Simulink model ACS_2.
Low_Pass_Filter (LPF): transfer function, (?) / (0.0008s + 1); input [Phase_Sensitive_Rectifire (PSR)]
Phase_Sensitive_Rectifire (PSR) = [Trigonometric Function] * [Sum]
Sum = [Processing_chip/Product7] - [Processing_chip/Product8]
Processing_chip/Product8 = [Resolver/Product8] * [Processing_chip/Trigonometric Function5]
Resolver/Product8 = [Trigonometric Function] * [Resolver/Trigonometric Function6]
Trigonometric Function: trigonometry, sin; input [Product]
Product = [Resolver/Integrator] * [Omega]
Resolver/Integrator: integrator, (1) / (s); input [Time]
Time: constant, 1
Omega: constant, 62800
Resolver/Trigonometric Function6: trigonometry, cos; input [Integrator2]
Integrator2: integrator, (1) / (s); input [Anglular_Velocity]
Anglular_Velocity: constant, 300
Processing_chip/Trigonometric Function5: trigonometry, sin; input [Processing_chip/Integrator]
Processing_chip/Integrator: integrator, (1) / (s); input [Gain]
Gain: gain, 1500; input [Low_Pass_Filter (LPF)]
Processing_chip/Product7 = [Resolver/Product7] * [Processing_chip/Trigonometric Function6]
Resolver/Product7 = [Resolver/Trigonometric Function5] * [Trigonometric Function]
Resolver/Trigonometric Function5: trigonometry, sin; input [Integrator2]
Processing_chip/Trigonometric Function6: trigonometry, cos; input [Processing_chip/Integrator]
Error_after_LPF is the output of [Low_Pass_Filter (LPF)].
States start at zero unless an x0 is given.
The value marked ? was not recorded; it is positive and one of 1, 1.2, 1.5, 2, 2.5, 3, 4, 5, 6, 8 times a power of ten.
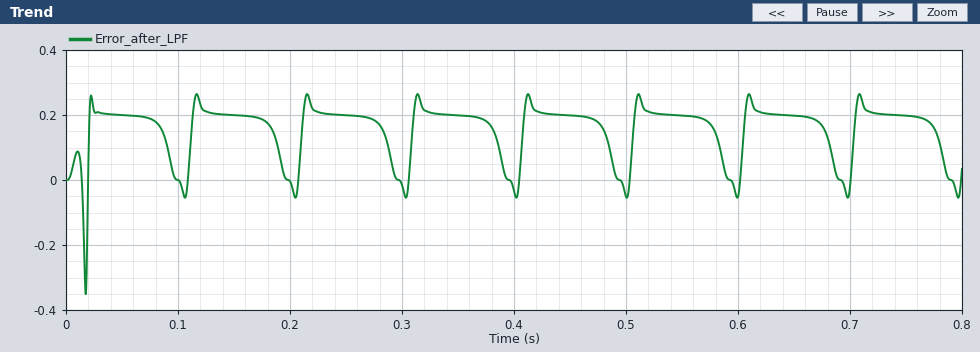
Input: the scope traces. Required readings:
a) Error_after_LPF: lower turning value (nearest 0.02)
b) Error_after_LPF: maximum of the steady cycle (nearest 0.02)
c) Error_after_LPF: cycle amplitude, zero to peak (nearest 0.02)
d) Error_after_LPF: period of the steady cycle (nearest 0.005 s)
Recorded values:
-0.06
0.26
0.16
0.100 s
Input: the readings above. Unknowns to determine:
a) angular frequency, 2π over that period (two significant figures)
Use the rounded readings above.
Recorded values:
63 rad/s
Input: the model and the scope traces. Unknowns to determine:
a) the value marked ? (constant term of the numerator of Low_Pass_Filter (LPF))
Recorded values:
1.5
